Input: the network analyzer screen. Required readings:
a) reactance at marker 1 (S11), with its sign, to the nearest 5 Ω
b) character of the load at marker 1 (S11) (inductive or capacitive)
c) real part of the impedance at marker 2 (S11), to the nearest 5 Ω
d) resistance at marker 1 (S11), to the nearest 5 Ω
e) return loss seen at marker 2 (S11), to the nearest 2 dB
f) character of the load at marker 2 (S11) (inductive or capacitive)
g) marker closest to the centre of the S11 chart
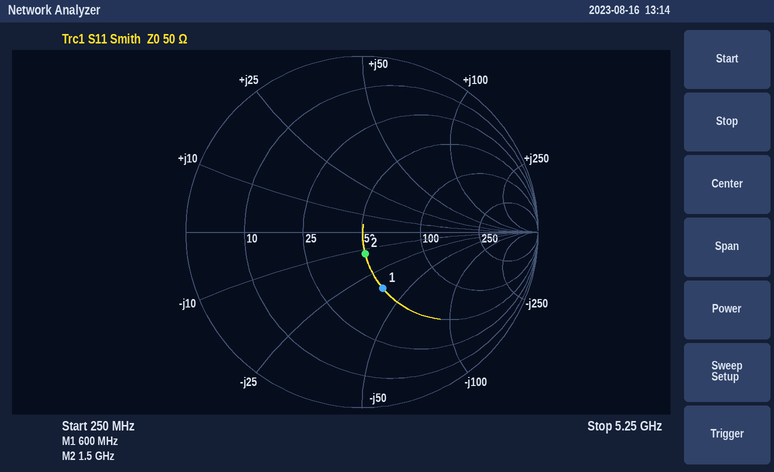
-35 Ω
capacitive
50 Ω
50 Ω
18 dB
capacitive
marker 2
